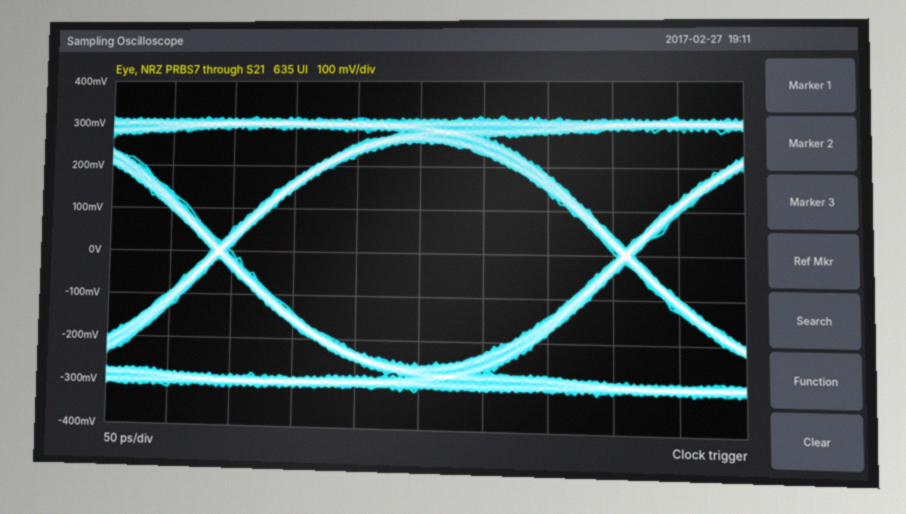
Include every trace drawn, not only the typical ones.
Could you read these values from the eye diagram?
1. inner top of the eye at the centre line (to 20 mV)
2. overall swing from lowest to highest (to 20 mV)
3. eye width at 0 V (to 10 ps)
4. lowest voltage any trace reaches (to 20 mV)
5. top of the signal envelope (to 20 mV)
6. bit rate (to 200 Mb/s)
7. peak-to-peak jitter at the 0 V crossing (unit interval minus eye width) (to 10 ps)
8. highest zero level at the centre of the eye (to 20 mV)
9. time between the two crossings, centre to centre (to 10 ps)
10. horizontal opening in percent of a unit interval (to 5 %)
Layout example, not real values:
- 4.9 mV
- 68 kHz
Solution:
- 260 mV
- 640 mV
- 300 ps
- -320 mV
- 320 mV
- 3.2 Gb/s
- 20 ps
- -260 mV
- 320 ps
- 95 %
